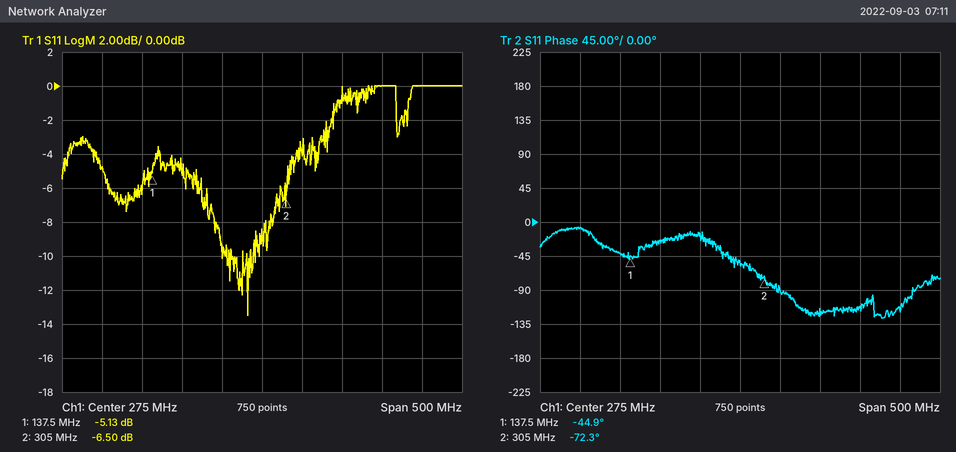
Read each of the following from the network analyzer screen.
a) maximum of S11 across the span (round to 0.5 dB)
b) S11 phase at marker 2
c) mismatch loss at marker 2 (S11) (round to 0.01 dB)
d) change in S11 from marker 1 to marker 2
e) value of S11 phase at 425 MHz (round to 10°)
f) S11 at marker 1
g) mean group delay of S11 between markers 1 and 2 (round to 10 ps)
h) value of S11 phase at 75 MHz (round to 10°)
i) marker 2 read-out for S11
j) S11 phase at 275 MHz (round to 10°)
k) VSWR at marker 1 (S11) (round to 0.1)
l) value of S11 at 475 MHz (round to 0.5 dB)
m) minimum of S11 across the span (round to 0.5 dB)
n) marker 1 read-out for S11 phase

0.0 dB
-72.3°
1.10 dB
-1.37 dB
-110°
-5.13 dB
450 ps
-10°
-6.50 dB
-50°
3.5
0.0 dB
-13.5 dB
-44.9°
